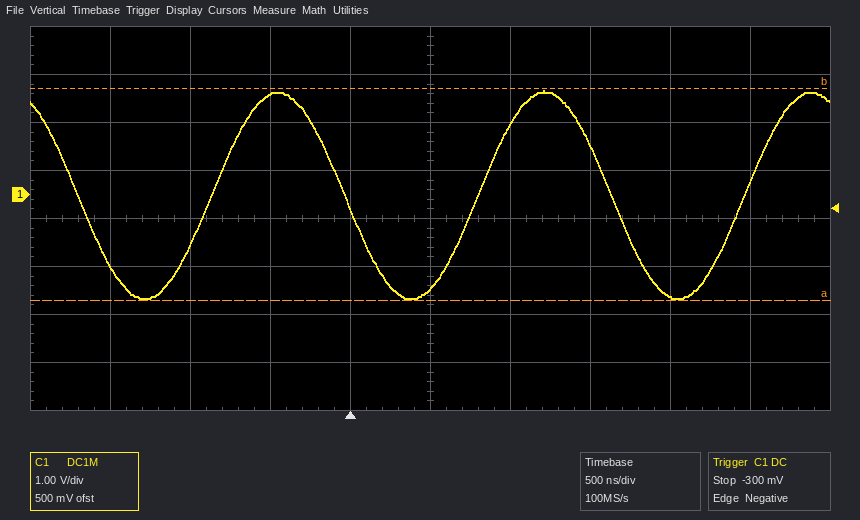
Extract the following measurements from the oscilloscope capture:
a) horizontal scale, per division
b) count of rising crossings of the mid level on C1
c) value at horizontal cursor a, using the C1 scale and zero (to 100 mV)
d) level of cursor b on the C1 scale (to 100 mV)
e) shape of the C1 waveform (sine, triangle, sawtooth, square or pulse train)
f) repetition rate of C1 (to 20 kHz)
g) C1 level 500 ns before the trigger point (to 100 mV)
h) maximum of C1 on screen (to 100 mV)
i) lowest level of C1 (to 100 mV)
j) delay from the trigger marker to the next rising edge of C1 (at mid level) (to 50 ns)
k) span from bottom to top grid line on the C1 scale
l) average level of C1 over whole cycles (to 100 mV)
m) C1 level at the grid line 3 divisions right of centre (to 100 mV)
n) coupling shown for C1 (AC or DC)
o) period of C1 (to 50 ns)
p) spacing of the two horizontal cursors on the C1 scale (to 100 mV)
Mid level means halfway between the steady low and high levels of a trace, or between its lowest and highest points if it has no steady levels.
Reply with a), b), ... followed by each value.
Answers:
a) 500 ns
b) 3
c) -2.2 V
d) 2.2 V
e) sine
f) 600 kHz
g) 2.1 V
h) 2.2 V
i) -2.2 V
j) 800 ns
k) 8 V
l) 0.0 V
m) -2.1 V
n) DC
o) 1.65 µs
p) 4.4 V
